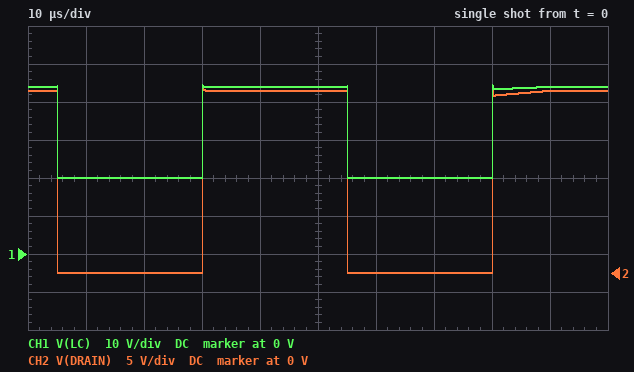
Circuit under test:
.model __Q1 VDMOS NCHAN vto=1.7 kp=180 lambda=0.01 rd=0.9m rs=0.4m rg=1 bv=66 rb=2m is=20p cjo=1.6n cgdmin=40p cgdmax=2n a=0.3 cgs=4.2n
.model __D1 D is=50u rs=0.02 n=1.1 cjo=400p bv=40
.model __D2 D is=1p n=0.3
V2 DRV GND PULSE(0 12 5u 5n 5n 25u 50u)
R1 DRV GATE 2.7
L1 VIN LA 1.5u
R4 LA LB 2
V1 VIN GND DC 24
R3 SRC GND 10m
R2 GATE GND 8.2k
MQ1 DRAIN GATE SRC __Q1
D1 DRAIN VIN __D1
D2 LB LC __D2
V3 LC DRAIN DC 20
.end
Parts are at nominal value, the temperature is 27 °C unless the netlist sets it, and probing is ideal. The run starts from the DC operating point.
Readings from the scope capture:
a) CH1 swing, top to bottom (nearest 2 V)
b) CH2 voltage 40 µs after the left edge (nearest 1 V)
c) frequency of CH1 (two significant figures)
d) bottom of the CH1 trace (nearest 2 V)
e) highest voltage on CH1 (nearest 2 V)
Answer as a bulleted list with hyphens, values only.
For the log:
- 24 V
- 24 V
- 20 kHz
- 20 V
- 44 V
